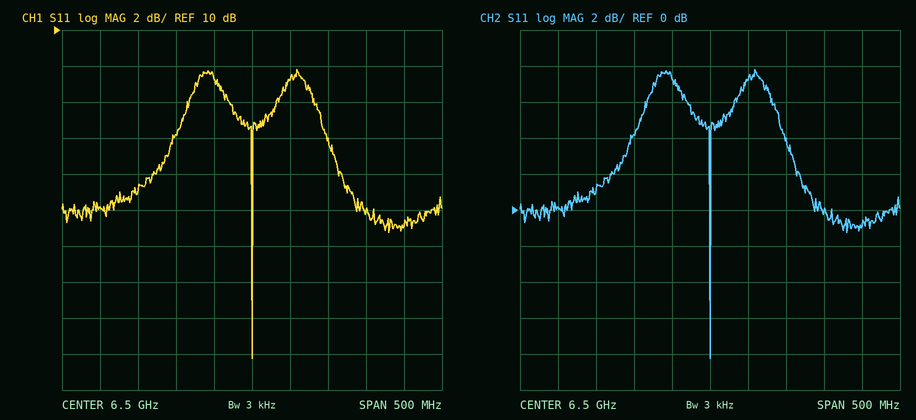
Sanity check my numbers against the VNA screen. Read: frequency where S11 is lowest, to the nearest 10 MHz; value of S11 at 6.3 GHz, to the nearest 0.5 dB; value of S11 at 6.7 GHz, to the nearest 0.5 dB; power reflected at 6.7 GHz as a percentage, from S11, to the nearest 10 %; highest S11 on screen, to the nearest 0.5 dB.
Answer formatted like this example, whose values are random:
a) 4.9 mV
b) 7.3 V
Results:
a) 6.50 GHz
b) 0.0 dB
c) -1.0 dB
d) 80 %
e) 8.0 dB
